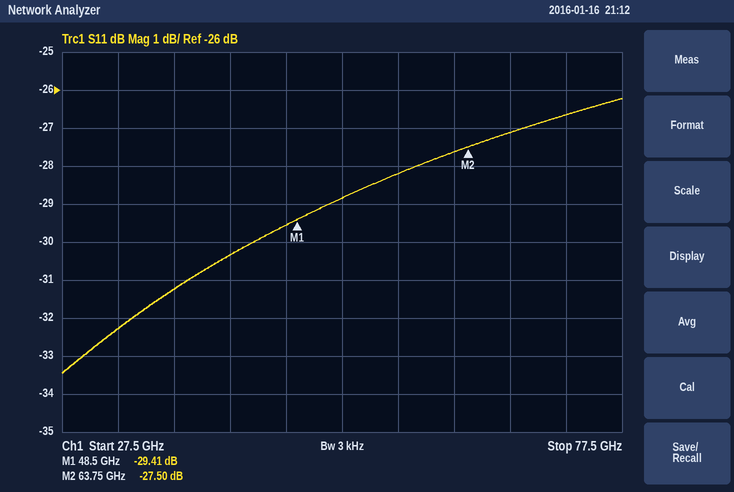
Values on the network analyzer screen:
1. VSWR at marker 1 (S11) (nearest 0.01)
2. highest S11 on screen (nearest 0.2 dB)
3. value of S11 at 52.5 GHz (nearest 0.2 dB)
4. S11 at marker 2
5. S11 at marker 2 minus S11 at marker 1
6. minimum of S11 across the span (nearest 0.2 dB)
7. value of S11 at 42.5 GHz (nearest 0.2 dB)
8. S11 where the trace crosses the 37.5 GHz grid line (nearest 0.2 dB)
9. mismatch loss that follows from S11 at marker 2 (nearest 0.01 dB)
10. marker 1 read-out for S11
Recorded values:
1.07
-26.2 dB
-28.8 dB
-27.50 dB
1.91 dB
-33.4 dB
-30.4 dB
-31.2 dB
0.01 dB
-29.41 dB
